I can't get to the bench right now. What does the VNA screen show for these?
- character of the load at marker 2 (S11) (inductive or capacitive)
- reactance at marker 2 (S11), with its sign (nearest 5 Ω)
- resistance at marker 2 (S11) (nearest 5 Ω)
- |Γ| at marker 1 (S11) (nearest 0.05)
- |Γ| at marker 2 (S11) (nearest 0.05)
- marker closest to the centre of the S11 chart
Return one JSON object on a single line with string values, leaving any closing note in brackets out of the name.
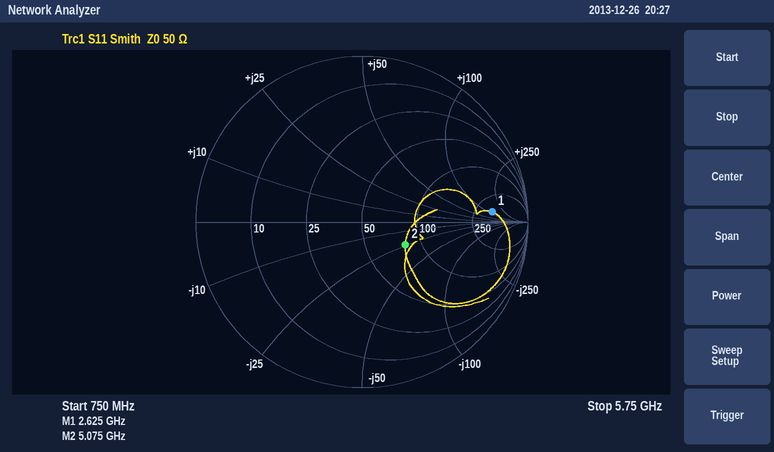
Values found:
{"character of the load at marker 2 (S11)": "capacitive", "reactance at marker 2 (S11), with its sign": "-25 Ω", "resistance at marker 2 (S11)": "80 Ω", "|Γ| at marker 1 (S11)": "0.80", "|Γ| at marker 2 (S11)": "0.30", "marker closest to the centre of the S11 chart": "marker 2"}
